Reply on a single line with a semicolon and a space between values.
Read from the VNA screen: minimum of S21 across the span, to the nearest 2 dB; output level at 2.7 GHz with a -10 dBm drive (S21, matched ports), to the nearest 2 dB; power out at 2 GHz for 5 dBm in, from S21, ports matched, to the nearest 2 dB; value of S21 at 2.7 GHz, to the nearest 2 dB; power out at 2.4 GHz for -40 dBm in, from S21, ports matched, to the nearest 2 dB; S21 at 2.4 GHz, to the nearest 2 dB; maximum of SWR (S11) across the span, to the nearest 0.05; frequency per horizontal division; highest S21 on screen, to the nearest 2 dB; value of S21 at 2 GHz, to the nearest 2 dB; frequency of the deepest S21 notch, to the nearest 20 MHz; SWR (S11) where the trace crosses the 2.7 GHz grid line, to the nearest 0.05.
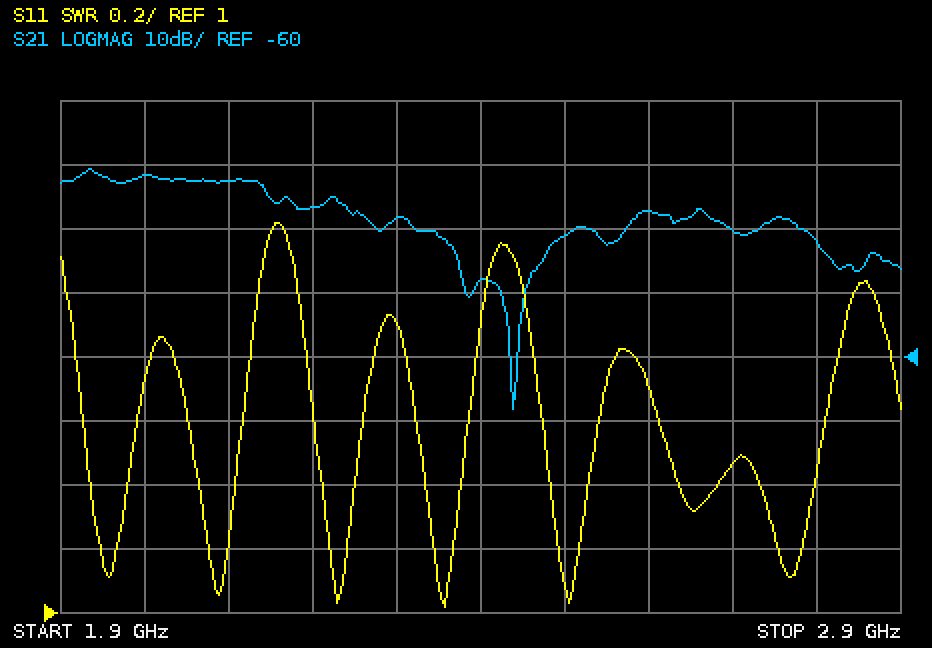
-68 dB; -50 dBm; -26 dBm; -40 dB; -88 dBm; -48 dB; 2.20; 100 MHz; -30 dB; -32 dB; 2.44 GHz; 1.45
